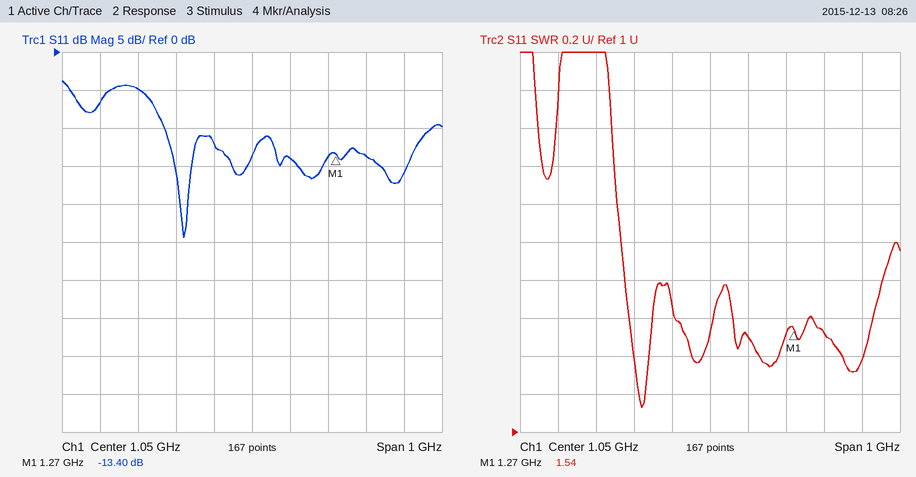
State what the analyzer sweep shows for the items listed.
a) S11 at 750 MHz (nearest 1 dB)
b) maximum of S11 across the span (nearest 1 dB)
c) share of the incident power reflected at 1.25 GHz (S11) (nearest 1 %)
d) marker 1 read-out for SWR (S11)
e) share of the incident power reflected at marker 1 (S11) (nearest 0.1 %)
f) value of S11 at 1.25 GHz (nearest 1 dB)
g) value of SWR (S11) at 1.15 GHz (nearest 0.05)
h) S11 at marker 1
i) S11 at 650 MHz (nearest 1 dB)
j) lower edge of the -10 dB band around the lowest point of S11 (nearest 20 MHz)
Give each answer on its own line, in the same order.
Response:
-5 dB
-4 dB
4 %
1.54
4.6 %
-14 dB
1.50
-13.40 dB
-7 dB
820 MHz
